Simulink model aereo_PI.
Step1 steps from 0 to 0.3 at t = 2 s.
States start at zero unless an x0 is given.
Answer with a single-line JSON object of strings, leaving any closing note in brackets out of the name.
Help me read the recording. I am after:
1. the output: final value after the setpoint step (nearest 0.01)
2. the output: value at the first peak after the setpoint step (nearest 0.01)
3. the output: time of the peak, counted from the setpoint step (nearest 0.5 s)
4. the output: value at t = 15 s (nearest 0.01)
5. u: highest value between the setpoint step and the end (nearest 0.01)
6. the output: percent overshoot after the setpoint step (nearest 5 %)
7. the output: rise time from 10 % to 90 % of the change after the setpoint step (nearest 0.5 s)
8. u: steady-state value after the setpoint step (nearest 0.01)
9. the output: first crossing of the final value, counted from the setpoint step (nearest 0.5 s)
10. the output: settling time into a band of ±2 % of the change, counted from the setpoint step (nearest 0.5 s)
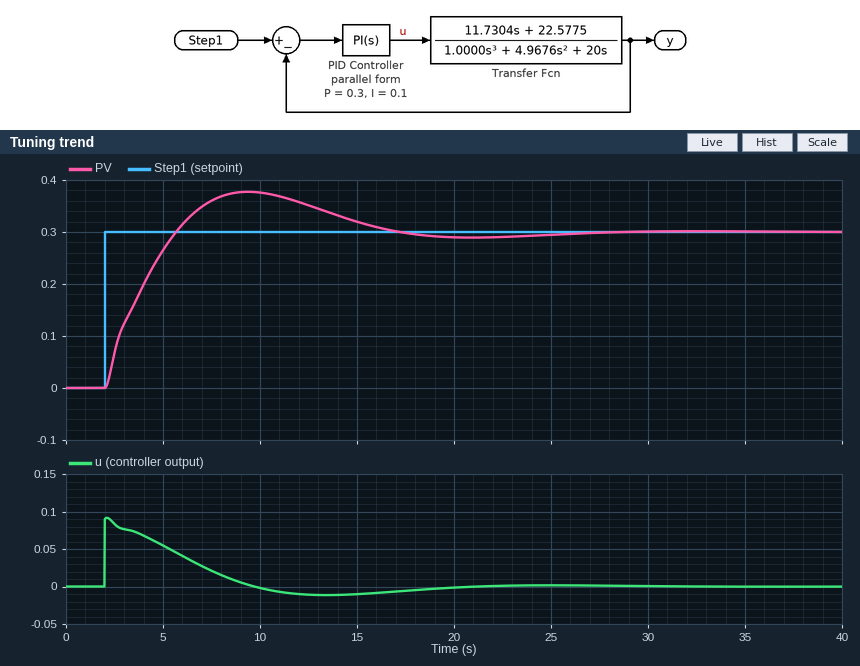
{"the output: final value after the setpoint step": "0.30", "the output: value at the first peak after the setpoint step": "0.38", "the output: time of the peak, counted from the setpoint step": "7.5 s", "the output: value at t = 15 s": "0.32", "u: highest value between the setpoint step and the end": "0.09", "the output: percent overshoot after the setpoint step": "25 %", "the output: rise time from 10 % to 90 % of the change after the setpoint step": "3.0 s", "u: steady-state value after the setpoint step": "0.00", "the output: first crossing of the final value, counted from the setpoint step": "3.5 s", "the output: settling time into a band of ±2 % of the change, counted from the setpoint step": "22.5 s"}
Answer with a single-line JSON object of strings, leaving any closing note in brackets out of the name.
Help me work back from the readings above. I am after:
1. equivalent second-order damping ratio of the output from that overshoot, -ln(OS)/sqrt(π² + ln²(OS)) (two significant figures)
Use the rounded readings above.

{"equivalent second-order damping ratio of the output from that overshoot, -ln(OS)/sqrt(π² + ln²(OS))": "0.40"}
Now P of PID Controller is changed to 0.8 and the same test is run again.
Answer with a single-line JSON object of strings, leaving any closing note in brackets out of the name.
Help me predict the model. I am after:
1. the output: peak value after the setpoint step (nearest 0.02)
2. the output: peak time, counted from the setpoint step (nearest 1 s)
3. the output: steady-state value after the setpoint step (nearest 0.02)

{"the output: peak value after the setpoint step": "0.32", "the output: peak time, counted from the setpoint step": "6 s", "the output: steady-state value after the setpoint step": "0.30"}
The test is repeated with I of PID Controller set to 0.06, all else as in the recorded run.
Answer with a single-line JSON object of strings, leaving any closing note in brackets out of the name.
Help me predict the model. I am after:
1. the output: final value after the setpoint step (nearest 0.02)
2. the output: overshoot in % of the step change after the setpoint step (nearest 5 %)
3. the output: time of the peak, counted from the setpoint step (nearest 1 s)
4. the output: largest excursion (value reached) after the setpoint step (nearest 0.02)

{"the output: final value after the setpoint step": "0.30", "the output: overshoot in % of the step change after the setpoint step": "20 %", "the output: time of the peak, counted from the setpoint step": "9 s", "the output: largest excursion (value reached) after the setpoint step": "0.36"}
